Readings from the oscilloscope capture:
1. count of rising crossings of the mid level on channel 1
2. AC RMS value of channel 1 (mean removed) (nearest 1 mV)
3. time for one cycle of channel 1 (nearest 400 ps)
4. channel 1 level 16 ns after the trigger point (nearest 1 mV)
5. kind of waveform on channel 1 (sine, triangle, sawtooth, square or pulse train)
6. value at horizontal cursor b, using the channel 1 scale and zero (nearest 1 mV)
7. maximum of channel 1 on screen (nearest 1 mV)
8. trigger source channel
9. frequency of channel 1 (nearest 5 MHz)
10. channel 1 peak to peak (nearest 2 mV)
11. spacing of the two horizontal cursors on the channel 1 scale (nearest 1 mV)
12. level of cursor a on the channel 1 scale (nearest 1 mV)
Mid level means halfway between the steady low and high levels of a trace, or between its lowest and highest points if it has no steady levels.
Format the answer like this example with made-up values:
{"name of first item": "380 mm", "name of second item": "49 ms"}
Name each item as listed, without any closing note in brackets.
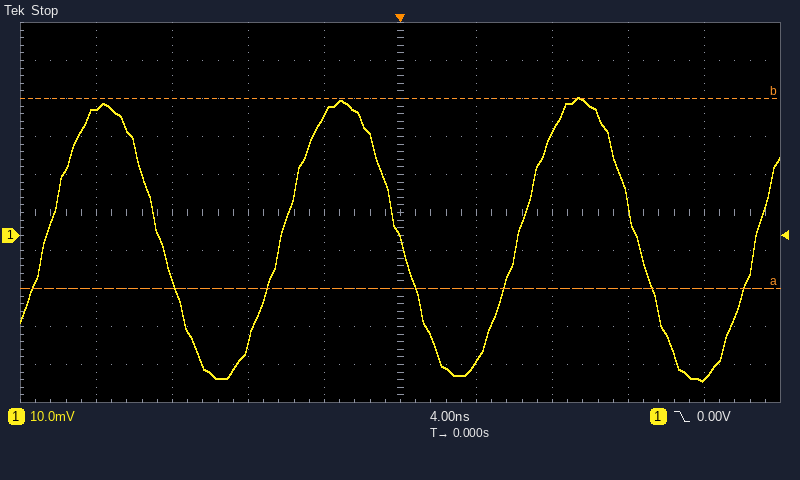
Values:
{"count of rising crossings of the mid level on channel 1": "4", "AC RMS value of channel 1 (mean removed)": "26 mV", "time for one cycle of channel 1": "12.4 ns", "channel 1 level 16 ns after the trigger point": "-38 mV", "kind of waveform on channel 1": "sine", "value at horizontal cursor b, using the channel 1 scale and zero": "36 mV", "maximum of channel 1 on screen": "36 mV", "trigger source channel": "channel 1", "frequency of channel 1": "80 MHz", "channel 1 peak to peak": "74 mV", "spacing of the two horizontal cursors on the channel 1 scale": "50 mV", "level of cursor a on the channel 1 scale": "-14 mV"}
